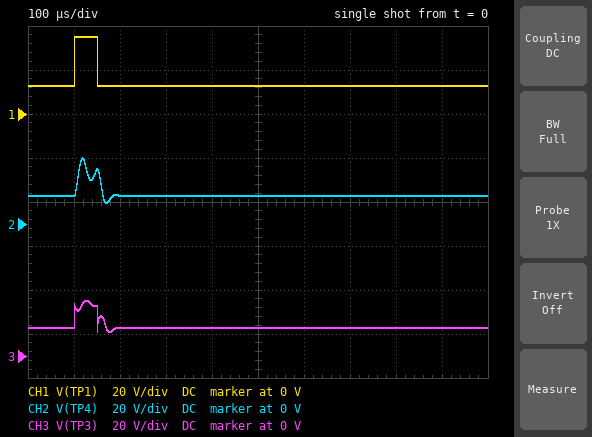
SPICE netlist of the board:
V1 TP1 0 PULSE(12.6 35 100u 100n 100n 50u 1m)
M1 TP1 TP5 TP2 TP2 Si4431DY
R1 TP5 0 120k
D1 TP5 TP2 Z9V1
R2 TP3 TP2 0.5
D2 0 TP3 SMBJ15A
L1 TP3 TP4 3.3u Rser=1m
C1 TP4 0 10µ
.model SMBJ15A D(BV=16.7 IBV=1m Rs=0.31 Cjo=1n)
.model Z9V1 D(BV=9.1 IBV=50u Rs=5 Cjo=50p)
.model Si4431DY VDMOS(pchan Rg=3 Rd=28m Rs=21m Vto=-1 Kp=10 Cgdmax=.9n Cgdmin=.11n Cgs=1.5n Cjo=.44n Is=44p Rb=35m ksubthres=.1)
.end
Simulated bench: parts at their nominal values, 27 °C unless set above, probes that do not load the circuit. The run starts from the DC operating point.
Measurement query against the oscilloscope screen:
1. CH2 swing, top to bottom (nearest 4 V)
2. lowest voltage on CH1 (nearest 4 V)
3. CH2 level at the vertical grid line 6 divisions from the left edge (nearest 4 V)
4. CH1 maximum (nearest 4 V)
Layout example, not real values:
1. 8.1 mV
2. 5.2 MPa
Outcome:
1. 20 V
2. 12 V
3. 12 V
4. 36 V
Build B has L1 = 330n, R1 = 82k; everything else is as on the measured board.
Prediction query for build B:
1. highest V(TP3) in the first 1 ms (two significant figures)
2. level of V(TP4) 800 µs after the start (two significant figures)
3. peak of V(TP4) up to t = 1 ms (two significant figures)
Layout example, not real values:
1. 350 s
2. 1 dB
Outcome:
1. 24 V
2. 13 V
3. 25 V
